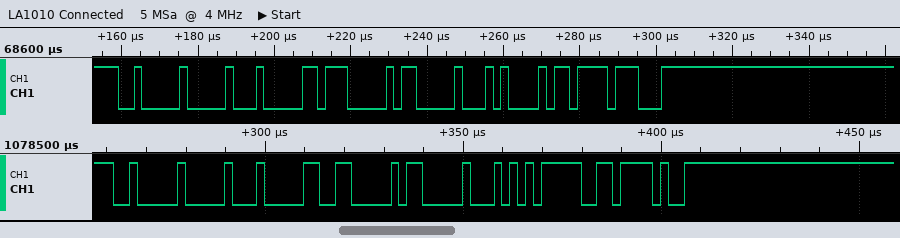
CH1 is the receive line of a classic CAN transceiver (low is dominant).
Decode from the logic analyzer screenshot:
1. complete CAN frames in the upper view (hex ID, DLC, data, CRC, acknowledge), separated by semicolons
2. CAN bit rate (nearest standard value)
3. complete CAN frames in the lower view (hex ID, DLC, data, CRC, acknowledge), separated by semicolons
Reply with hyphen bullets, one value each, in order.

- ID 200, DLC 4, data 17 03 00 A1, CRC 37B8, NACK
- 500 kbit/s
- ID 200, DLC 4, data 13 03 00 AB, CRC 76F4, NACK
